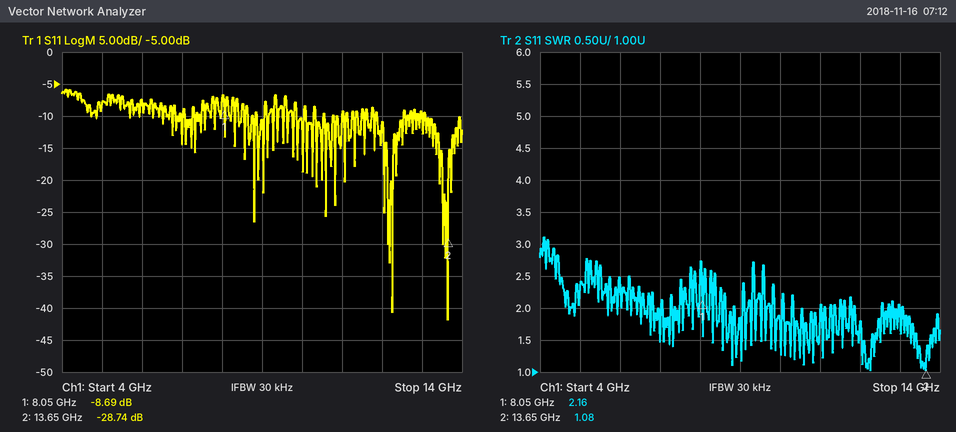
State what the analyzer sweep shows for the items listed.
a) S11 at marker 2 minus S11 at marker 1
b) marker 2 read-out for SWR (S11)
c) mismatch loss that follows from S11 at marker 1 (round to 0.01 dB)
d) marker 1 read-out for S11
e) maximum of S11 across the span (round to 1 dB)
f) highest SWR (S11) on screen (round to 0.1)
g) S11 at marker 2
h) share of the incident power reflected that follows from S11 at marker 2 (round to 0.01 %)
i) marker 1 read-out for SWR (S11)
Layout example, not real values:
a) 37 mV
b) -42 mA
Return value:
a) -20.05 dB
b) 1.08
c) 0.63 dB
d) -8.69 dB
e) -6 dB
f) 3.1
g) -28.74 dB
h) 0.13 %
i) 2.16
